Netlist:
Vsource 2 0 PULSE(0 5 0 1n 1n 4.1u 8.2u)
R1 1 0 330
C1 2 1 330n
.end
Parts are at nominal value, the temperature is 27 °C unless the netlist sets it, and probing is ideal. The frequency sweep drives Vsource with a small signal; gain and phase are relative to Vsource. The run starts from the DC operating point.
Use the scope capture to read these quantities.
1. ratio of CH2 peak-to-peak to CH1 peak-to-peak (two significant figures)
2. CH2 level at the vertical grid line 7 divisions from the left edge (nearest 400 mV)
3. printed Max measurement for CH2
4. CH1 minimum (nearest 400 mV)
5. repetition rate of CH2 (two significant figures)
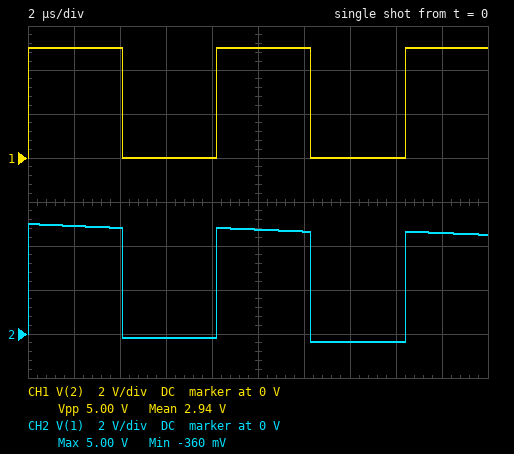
1.1
-400 mV
5.00 V
0 V
120 kHz
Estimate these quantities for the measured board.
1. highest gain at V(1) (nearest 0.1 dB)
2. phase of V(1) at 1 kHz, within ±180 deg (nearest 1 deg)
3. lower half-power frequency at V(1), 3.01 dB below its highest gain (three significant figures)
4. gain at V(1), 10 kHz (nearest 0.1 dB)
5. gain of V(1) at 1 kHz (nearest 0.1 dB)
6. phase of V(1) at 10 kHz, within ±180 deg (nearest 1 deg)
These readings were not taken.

0 dB
56 deg
1.46 kHz
-0.1 dB
-5.0 dB
8 deg
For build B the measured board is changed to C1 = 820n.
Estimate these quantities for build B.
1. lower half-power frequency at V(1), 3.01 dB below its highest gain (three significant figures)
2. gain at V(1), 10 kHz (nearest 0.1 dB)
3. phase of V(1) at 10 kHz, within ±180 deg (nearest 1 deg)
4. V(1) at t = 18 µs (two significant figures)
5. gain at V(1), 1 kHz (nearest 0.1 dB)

588 Hz
0 dB
3 deg
4.8 V
-1.3 dB
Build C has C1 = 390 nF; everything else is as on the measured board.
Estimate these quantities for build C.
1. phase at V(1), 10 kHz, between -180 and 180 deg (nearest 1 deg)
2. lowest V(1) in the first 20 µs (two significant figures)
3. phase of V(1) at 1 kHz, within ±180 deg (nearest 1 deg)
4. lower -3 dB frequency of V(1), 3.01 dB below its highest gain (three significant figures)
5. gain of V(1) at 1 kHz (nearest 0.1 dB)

7 deg
-300 mV
51 deg
1.24 kHz
-4.0 dB
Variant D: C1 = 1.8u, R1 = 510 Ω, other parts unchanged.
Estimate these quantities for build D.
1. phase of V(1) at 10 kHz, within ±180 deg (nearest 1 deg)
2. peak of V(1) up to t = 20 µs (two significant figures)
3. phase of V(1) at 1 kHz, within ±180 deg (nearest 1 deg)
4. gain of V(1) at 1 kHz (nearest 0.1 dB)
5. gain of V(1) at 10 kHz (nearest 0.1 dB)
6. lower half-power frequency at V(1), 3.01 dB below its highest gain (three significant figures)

1 deg
5.0 V
10 deg
-0.1 dB
0 dB
173 Hz
